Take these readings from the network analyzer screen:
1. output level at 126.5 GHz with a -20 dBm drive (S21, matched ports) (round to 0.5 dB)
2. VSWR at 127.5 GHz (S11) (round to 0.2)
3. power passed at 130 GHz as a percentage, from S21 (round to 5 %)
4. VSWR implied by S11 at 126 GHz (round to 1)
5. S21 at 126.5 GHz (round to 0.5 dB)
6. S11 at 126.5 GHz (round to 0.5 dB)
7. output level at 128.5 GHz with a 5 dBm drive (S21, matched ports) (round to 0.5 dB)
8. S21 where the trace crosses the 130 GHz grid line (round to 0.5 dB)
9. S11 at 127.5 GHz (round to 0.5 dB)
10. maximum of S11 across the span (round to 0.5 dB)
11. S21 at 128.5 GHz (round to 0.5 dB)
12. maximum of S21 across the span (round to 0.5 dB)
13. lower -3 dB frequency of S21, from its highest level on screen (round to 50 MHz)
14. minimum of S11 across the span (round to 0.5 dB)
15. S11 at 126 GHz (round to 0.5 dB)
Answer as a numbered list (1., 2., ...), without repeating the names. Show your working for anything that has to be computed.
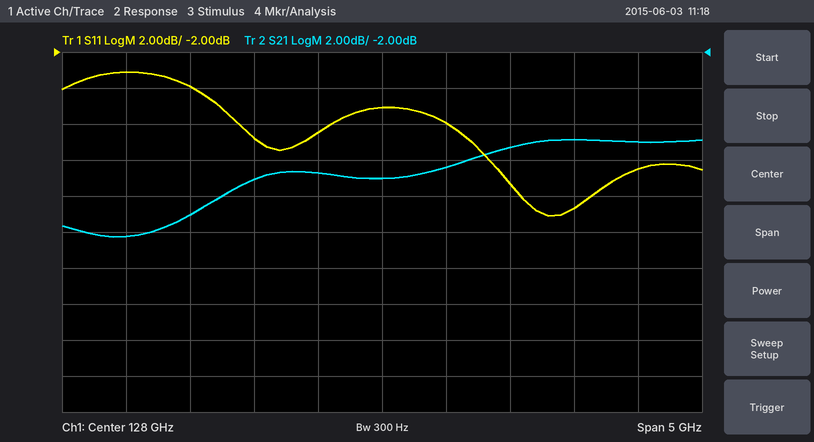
1. -20 dBm + (-11.0 dB) = -31.0 dBm
2. |Γ| = 10^(-6.5/20) = 0.4732; VSWR = (1 + 0.4732)/(1 − 0.4732) ≈ 2.8
3. 10^(-7/10) ≈ 20 %
4. |Γ| = 10^(-3/20) = 0.7079; VSWR = (1 + 0.7079)/(1 − 0.7079) ≈ 6
5. -11.0 dB
6. -4.0 dB
7. 5 dBm + (-8.5 dB) = -3.5 dBm
8. -7.0 dB
9. -6.5 dB
10. -3.0 dB
11. -8.5 dB
12. -7.0 dB
13. 126.80 GHz
14. -11.0 dB
15. -3.0 dB
